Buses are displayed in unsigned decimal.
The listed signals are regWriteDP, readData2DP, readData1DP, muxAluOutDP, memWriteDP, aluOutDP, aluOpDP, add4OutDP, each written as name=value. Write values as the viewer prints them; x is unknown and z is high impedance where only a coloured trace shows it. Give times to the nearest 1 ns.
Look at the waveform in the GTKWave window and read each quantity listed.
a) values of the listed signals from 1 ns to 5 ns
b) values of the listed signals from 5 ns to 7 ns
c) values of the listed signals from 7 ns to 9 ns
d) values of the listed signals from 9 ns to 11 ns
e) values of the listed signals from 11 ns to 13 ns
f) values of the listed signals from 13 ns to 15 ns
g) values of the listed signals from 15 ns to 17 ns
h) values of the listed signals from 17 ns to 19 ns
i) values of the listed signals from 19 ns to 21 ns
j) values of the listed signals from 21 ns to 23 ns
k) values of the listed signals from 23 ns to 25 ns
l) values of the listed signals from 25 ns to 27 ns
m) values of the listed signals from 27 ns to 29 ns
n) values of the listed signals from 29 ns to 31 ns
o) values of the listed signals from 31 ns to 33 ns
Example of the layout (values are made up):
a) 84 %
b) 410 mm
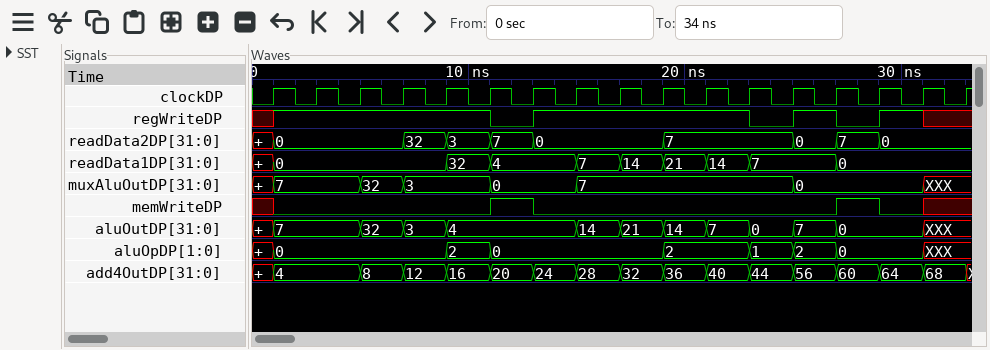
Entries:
a) regWriteDP=1, readData2DP=0, readData1DP=0, muxAluOutDP=7, memWriteDP=0, aluOutDP=7, aluOpDP=0, add4OutDP=4
b) regWriteDP=1, readData2DP=0, readData1DP=0, muxAluOutDP=32, memWriteDP=0, aluOutDP=32, aluOpDP=0, add4OutDP=8
c) regWriteDP=1, readData2DP=32, readData1DP=0, muxAluOutDP=3, memWriteDP=0, aluOutDP=3, aluOpDP=0, add4OutDP=12
d) regWriteDP=1, readData2DP=3, readData1DP=32, muxAluOutDP=3, memWriteDP=0, aluOutDP=4, aluOpDP=2, add4OutDP=16
e) regWriteDP=0, readData2DP=7, readData1DP=4, muxAluOutDP=0, memWriteDP=1, aluOutDP=4, aluOpDP=0, add4OutDP=20
f) regWriteDP=1, readData2DP=0, readData1DP=4, muxAluOutDP=0, memWriteDP=0, aluOutDP=4, aluOpDP=0, add4OutDP=24
g) regWriteDP=1, readData2DP=0, readData1DP=7, muxAluOutDP=7, memWriteDP=0, aluOutDP=14, aluOpDP=0, add4OutDP=28
h) regWriteDP=1, readData2DP=0, readData1DP=14, muxAluOutDP=7, memWriteDP=0, aluOutDP=21, aluOpDP=0, add4OutDP=32
i) regWriteDP=1, readData2DP=7, readData1DP=21, muxAluOutDP=7, memWriteDP=0, aluOutDP=14, aluOpDP=2, add4OutDP=36
j) regWriteDP=1, readData2DP=7, readData1DP=14, muxAluOutDP=7, memWriteDP=0, aluOutDP=7, aluOpDP=2, add4OutDP=40
k) regWriteDP=0, readData2DP=7, readData1DP=7, muxAluOutDP=7, memWriteDP=0, aluOutDP=0, aluOpDP=1, add4OutDP=44
l) regWriteDP=1, readData2DP=0, readData1DP=7, muxAluOutDP=0, memWriteDP=0, aluOutDP=7, aluOpDP=2, add4OutDP=56
m) regWriteDP=0, readData2DP=7, readData1DP=0, muxAluOutDP=0, memWriteDP=1, aluOutDP=0, aluOpDP=0, add4OutDP=60
n) regWriteDP=1, readData2DP=0, readData1DP=0, muxAluOutDP=0, memWriteDP=0, aluOutDP=0, aluOpDP=0, add4OutDP=64
o) regWriteDP=x, readData2DP=0, readData1DP=0, muxAluOutDP=XXX, memWriteDP=x, aluOutDP=XXX, aluOpDP=XXX, add4OutDP=68
